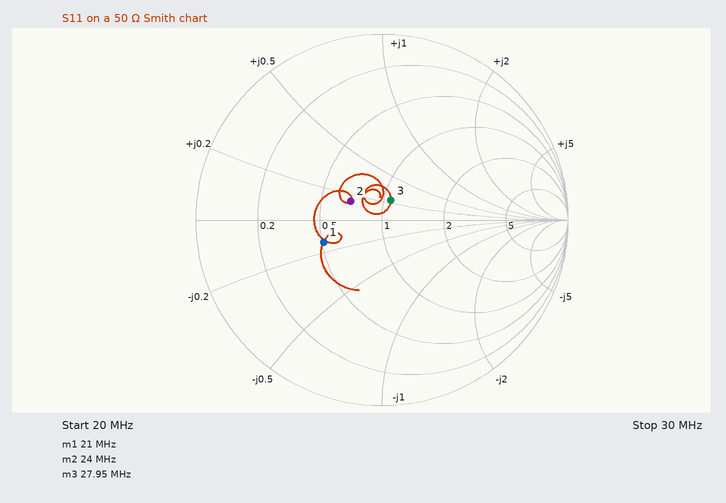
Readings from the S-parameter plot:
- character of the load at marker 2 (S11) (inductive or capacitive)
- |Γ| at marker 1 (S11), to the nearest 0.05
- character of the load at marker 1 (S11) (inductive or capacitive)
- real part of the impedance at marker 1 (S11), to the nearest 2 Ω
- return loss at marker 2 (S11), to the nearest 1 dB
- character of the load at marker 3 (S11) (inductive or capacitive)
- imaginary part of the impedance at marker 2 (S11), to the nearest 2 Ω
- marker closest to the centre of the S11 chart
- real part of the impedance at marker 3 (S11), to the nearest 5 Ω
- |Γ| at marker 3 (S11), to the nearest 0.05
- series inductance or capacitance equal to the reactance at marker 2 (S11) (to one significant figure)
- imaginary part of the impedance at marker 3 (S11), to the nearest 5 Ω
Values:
inductive
0.35
capacitive
26 Ω
14 dB
inductive
+8 Ω
marker 3
55 Ω
0.10
50 nH
+10 Ω
